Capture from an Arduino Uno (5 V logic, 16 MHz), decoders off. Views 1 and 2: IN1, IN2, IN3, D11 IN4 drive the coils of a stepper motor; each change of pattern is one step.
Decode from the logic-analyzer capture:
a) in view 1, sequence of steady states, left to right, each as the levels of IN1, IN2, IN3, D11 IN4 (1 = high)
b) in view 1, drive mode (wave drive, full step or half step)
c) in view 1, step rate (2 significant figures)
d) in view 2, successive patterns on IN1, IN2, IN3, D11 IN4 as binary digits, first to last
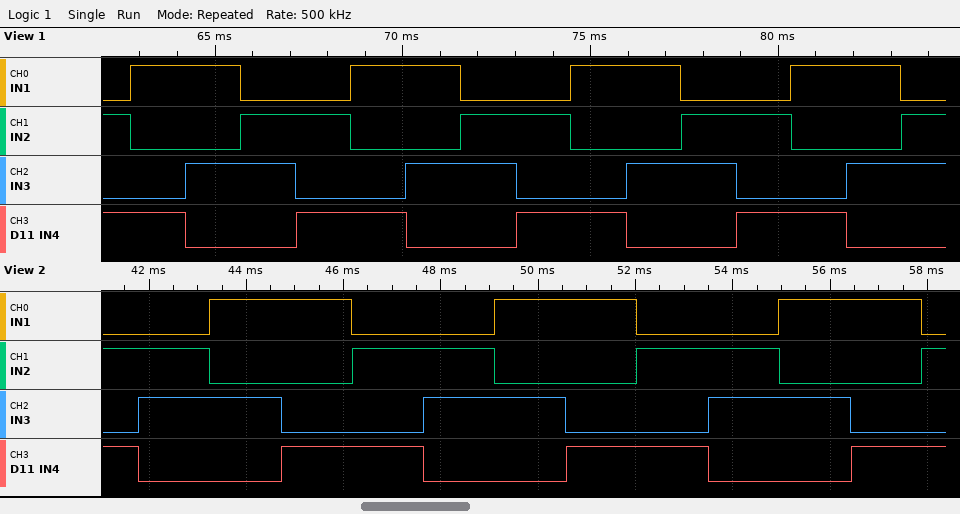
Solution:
0101 1001 1010 0110 0101 1001 1010 0110 0101 1001 1010 0110 0101 1001 1010 0110
full step
680 steps/s
0101 0110 1010 1001 0101 0110 1010 1001 0101 0110 1010 1001 0101
